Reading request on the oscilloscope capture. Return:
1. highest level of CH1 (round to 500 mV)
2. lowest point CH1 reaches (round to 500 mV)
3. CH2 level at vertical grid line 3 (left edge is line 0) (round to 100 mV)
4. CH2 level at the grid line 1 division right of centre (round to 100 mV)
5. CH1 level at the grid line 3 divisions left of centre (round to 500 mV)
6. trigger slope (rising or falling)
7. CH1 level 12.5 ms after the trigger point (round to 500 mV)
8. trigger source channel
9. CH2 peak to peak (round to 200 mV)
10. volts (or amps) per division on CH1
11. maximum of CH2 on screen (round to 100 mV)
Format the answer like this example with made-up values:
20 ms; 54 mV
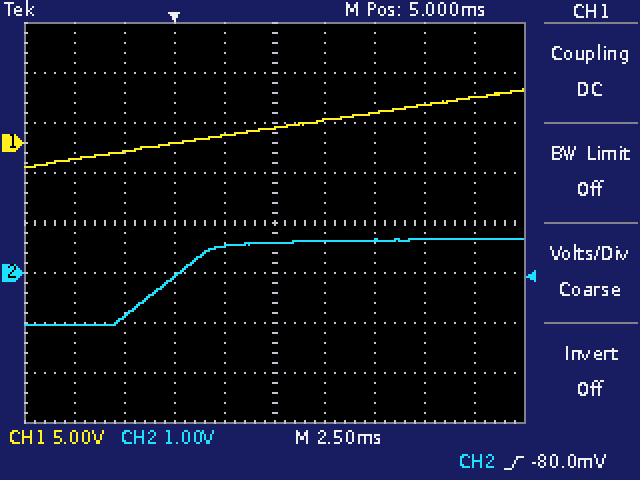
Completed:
5.5 V; -2.5 V; -100 mV; 600 mV; -1.0 V; rising; 4.0 V; CH2; 1.8 V; 5 V; 700 mV
